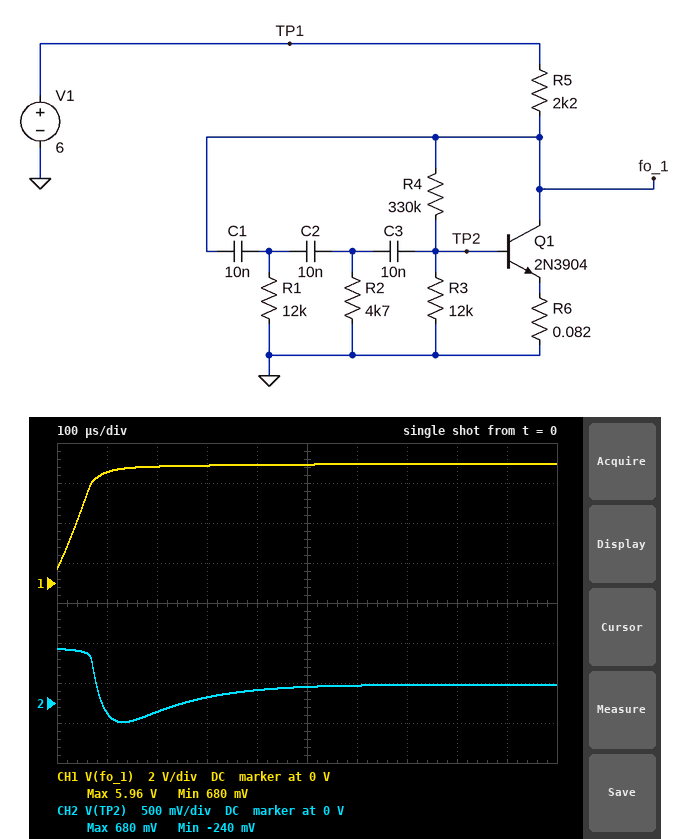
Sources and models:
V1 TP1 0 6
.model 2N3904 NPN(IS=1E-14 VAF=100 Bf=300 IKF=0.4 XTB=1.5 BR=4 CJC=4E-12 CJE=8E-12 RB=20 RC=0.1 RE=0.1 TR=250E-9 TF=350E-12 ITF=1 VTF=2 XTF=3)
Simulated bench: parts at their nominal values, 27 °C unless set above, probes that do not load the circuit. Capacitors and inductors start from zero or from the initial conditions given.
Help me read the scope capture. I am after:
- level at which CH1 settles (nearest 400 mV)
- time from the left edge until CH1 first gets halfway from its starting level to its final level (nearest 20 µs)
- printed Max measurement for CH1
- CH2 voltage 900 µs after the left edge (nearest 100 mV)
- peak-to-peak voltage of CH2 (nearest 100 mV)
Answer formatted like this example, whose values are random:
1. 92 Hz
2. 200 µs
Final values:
1. 6.0 V
2. 40 µs
3. 5.96 V
4. 200 mV
5. 900 mV
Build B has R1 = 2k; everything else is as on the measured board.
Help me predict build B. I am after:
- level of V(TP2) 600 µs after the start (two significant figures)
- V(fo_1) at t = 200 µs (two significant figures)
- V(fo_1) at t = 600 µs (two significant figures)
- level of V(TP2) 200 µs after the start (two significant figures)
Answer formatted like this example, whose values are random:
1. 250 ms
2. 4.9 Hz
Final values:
1. 210 mV
2. 5.9 V
3. 6.0 V
4. 110 mV
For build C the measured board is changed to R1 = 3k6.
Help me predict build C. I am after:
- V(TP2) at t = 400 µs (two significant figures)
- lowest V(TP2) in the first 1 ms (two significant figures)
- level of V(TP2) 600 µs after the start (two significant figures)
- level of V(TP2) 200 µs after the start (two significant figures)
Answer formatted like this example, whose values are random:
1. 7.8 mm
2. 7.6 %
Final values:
1. 210 mV
2. -270 mV
3. 220 mV
4. 30 mV
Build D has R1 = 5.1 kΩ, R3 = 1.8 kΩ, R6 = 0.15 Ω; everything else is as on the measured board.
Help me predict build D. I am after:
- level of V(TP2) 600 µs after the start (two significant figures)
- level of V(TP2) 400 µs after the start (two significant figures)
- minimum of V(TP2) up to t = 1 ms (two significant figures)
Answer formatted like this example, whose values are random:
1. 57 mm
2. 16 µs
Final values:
1. 35 mV
2. 40 mV
3. -200 mV
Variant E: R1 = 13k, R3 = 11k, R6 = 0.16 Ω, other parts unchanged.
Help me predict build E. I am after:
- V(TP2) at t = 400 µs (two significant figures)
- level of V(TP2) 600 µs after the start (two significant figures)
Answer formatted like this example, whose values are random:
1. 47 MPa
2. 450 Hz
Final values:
1. 150 mV
2. 200 mV
